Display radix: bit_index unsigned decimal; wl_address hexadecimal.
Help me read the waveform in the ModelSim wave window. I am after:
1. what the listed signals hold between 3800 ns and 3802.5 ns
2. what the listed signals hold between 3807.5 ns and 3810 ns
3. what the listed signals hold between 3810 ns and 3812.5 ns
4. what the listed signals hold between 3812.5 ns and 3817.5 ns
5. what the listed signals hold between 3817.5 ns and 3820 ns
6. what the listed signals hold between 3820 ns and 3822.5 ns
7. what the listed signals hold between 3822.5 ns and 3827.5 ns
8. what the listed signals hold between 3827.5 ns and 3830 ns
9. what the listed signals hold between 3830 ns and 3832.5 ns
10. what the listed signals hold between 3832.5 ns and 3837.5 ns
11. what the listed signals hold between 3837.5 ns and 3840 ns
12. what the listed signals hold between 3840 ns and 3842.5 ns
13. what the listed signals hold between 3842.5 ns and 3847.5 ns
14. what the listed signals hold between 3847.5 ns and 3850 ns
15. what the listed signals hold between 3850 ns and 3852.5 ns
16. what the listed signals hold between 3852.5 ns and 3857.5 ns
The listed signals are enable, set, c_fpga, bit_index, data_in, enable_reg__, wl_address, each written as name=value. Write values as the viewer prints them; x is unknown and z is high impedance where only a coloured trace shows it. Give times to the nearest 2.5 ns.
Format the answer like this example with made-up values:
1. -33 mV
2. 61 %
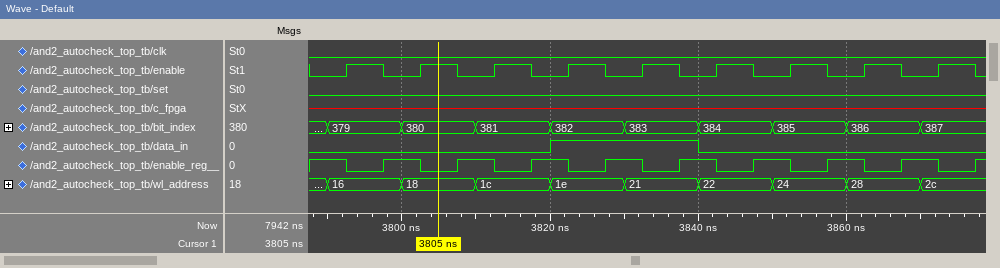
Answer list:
1. enable=0, set=0, c_fpga=x, bit_index=380, data_in=0, enable_reg__=1, wl_address=18
2. enable=0, set=0, c_fpga=x, bit_index=380, data_in=0, enable_reg__=1, wl_address=18
3. enable=0, set=0, c_fpga=x, bit_index=381, data_in=0, enable_reg__=1, wl_address=1c
4. enable=1, set=0, c_fpga=x, bit_index=381, data_in=0, enable_reg__=0, wl_address=1c
5. enable=0, set=0, c_fpga=x, bit_index=381, data_in=0, enable_reg__=1, wl_address=1c
6. enable=0, set=0, c_fpga=x, bit_index=382, data_in=1, enable_reg__=1, wl_address=1e
7. enable=1, set=0, c_fpga=x, bit_index=382, data_in=1, enable_reg__=0, wl_address=1e
8. enable=0, set=0, c_fpga=x, bit_index=382, data_in=1, enable_reg__=1, wl_address=1e
9. enable=0, set=0, c_fpga=x, bit_index=383, data_in=1, enable_reg__=1, wl_address=21
10. enable=1, set=0, c_fpga=x, bit_index=383, data_in=1, enable_reg__=0, wl_address=21
11. enable=0, set=0, c_fpga=x, bit_index=383, data_in=1, enable_reg__=1, wl_address=21
12. enable=0, set=0, c_fpga=x, bit_index=384, data_in=0, enable_reg__=1, wl_address=22
13. enable=1, set=0, c_fpga=x, bit_index=384, data_in=0, enable_reg__=0, wl_address=22
14. enable=0, set=0, c_fpga=x, bit_index=384, data_in=0, enable_reg__=1, wl_address=22
15. enable=0, set=0, c_fpga=x, bit_index=385, data_in=0, enable_reg__=1, wl_address=24
16. enable=1, set=0, c_fpga=x, bit_index=385, data_in=0, enable_reg__=0, wl_address=24
